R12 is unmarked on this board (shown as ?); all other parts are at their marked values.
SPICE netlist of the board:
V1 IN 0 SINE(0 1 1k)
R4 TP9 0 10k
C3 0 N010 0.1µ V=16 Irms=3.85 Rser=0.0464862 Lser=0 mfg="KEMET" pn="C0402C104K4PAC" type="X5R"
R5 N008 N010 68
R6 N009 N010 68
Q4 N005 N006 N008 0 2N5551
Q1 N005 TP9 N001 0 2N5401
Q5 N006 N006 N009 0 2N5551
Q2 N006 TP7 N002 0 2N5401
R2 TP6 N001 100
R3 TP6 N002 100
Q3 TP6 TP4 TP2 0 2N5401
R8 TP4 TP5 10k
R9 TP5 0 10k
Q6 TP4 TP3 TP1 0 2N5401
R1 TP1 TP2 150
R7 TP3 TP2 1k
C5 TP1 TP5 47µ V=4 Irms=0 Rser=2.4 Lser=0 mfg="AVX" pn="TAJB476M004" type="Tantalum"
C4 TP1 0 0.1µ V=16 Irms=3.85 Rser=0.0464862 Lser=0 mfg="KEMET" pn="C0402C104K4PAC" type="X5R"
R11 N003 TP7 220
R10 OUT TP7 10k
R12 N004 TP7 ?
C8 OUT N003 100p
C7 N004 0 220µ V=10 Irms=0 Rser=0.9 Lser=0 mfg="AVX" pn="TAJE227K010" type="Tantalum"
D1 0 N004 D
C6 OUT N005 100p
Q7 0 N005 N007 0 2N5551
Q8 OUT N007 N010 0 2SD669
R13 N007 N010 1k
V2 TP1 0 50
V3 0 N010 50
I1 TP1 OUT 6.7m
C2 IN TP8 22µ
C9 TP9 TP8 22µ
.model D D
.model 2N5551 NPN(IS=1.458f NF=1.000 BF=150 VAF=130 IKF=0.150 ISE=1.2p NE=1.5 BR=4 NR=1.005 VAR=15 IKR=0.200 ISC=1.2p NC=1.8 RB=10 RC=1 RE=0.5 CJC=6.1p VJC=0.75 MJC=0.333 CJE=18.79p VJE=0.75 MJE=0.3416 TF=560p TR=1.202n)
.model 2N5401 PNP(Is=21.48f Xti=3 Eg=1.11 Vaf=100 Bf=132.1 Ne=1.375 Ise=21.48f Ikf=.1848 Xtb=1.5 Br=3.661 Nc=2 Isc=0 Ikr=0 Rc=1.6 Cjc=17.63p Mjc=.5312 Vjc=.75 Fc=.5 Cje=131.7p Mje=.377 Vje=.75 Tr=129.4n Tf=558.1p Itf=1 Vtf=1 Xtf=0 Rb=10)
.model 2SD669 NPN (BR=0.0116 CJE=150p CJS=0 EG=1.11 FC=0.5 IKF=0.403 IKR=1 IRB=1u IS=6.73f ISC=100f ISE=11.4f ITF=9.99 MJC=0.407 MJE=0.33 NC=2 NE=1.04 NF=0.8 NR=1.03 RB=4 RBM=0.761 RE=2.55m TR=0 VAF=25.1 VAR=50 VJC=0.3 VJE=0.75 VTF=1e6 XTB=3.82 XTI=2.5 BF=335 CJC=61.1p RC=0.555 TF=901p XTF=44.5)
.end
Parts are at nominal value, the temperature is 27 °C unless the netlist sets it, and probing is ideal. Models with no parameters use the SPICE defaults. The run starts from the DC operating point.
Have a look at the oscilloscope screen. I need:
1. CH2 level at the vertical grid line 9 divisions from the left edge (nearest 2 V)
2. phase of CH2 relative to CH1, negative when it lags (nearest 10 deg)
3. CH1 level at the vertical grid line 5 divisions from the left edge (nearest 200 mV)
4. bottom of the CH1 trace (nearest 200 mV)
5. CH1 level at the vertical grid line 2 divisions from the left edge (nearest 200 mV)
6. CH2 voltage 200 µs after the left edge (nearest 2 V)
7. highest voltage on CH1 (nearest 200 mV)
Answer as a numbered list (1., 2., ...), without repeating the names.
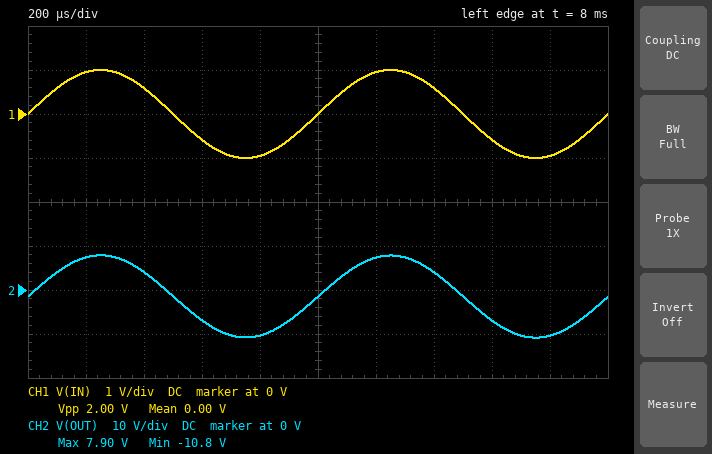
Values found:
1. -10 V
2. 0 deg
3. 0 V
4. -1.0 V
5. 600 mV
6. 8 V
7. 1.0 V
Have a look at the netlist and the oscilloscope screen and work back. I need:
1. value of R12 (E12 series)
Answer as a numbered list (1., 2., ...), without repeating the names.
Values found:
1. 1.2 kΩ
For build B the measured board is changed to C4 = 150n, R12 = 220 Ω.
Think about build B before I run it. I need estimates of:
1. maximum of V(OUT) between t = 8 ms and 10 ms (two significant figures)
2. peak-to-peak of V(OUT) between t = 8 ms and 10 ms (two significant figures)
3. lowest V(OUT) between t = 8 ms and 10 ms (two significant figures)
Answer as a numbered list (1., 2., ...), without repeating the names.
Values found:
1. 39 V
2. 89 V
3. -50 V
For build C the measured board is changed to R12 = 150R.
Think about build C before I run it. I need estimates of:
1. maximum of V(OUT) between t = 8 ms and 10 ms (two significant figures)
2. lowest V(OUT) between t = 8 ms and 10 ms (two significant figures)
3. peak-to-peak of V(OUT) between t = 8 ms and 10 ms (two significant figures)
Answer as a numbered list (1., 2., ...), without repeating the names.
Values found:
1. 57 V
2. -50 V
3. 110 V
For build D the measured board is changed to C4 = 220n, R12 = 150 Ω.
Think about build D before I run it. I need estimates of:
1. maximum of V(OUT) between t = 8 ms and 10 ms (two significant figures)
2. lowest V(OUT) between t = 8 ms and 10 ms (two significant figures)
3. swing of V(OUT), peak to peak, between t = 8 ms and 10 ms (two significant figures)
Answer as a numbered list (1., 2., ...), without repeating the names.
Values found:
1. 57 V
2. -50 V
3. 110 V
